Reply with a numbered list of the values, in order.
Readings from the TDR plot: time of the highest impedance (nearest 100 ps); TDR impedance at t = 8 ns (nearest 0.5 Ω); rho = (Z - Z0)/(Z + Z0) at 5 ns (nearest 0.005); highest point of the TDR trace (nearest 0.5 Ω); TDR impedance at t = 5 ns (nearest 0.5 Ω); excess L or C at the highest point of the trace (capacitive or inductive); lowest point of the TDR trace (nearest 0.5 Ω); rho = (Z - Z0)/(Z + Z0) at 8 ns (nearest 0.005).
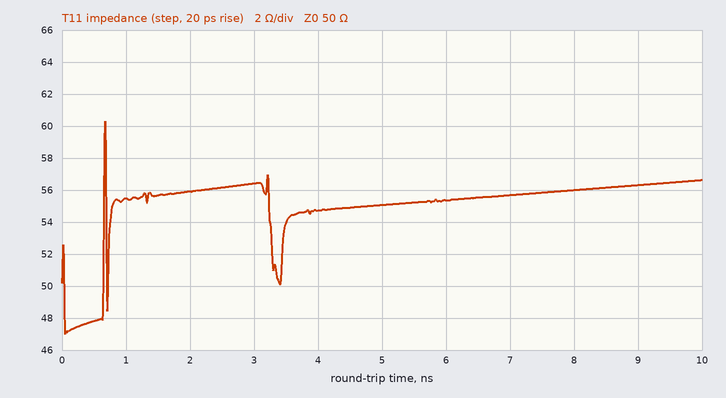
1. 700 ps
2. 56.0 Ω
3. +0.050
4. 60.5 Ω
5. 55.0 Ω
6. inductive
7. 47.0 Ω
8. +0.055
